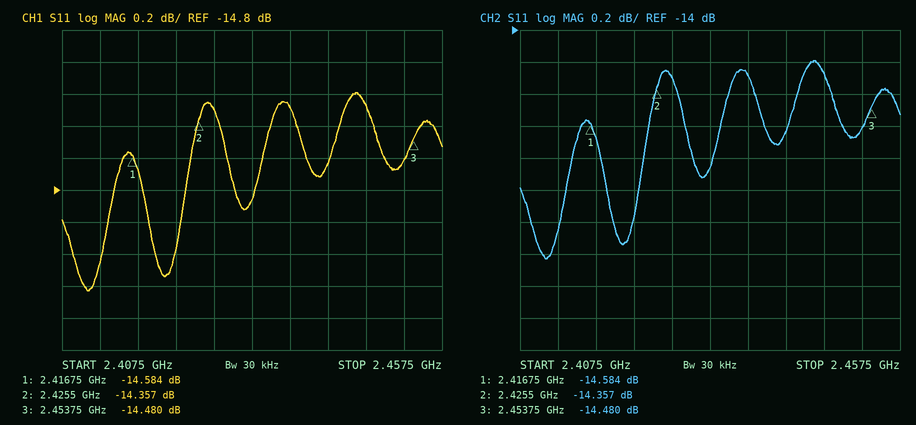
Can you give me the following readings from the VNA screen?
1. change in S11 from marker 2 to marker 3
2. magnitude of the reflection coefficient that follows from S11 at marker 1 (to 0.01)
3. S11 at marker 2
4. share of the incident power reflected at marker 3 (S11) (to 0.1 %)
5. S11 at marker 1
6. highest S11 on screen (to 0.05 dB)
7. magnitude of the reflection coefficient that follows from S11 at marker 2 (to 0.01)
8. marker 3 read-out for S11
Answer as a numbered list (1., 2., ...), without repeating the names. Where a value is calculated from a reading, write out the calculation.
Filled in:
1. -14.48 − (-14.357) = -0.123 dB
2. 10^(-14.584/20) ≈ 0.19
3. -14.357 dB
4. 10^(-14.48/10) ≈ 3.6 %
5. -14.584 dB
6. -14.20 dB
7. 10^(-14.357/20) ≈ 0.19
8. -14.480 dB
